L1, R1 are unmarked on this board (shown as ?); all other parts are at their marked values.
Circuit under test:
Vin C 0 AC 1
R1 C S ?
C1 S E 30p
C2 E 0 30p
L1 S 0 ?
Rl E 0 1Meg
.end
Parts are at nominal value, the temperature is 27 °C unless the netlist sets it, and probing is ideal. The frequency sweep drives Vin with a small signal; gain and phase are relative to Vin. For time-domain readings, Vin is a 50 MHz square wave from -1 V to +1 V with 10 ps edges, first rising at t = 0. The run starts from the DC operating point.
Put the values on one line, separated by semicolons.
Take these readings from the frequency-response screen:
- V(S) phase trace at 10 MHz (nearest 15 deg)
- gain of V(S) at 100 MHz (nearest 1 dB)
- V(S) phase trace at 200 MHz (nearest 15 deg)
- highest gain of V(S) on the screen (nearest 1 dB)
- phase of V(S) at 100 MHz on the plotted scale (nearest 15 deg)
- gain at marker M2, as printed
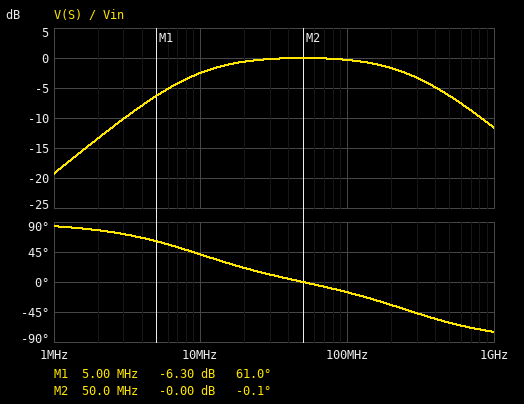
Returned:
45 deg; 0 dB; -30 deg; 0 dB; -15 deg; -0.00 dB
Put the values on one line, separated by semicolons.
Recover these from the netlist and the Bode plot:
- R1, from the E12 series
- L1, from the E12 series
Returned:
39 Ω; 680 nH
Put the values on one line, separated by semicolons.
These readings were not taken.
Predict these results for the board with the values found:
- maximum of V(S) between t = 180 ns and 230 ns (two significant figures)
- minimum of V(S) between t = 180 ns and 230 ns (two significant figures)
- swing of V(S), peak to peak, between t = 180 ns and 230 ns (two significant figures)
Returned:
1.2 V; -1.2 V; 2.3 V
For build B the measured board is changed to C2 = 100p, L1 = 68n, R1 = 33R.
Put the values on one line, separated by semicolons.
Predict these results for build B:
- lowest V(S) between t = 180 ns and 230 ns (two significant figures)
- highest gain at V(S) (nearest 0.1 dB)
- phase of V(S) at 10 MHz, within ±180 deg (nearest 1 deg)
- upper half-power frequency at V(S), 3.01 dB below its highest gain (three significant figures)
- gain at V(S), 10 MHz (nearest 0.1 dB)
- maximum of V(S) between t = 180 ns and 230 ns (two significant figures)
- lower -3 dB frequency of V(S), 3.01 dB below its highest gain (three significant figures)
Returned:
-1.4 V; 0 dB; 83 deg; 269 MHz; -17.8 dB; 1.4 V; 60.0 MHz
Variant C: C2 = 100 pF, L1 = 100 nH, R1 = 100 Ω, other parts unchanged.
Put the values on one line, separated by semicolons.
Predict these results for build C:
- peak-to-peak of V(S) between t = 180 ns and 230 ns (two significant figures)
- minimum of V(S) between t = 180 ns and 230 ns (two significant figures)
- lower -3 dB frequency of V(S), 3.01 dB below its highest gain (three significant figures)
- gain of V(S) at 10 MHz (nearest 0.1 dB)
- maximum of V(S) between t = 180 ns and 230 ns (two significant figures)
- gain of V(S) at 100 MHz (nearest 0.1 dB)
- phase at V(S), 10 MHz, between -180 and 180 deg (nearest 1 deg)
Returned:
1.5 V; -770 mV; 75.8 MHz; -24.0 dB; 770 mV; -0.1 dB; 86 deg
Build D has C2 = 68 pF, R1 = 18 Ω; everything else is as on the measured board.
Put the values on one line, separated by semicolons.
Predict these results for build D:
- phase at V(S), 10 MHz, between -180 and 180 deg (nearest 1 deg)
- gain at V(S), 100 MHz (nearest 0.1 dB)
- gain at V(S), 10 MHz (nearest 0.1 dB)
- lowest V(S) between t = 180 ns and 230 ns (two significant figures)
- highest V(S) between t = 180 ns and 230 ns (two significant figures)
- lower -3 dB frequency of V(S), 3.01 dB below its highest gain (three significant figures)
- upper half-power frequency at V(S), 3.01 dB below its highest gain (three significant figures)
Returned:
22 deg; -0.2 dB; -0.6 dB; -1.1 V; 1.1 V; 4.17 MHz; 429 MHz
